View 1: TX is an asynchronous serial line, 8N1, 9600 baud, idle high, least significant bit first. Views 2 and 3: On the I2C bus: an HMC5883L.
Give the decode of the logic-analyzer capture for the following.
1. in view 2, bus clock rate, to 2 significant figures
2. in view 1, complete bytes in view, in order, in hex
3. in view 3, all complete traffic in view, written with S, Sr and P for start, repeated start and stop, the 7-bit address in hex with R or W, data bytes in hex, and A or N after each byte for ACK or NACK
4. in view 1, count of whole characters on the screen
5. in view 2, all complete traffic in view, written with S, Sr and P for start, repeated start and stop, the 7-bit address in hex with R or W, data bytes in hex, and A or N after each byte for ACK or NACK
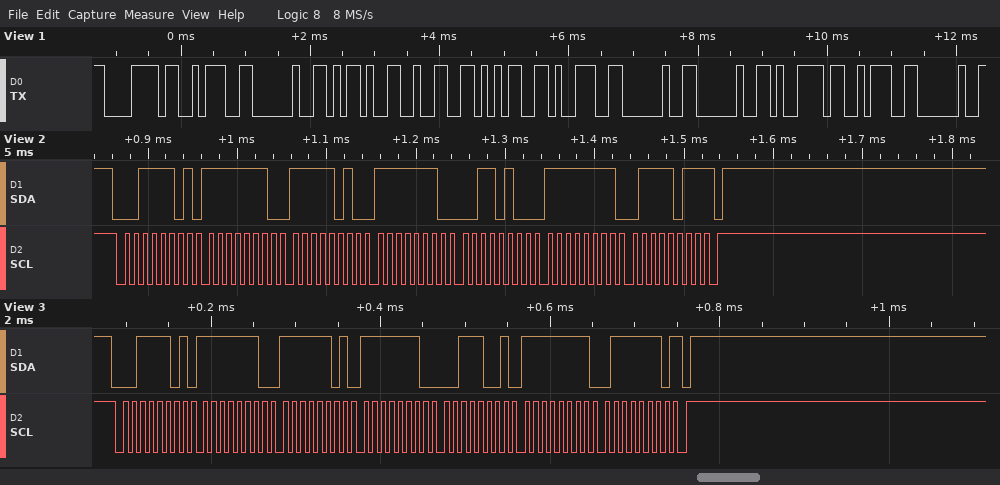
100 kHz
78 3A 20 2D 32 35 39 20 20 79 3A 20
S 1ER A FE A FD A FE A 39 A FF A 7E N P
12
S 1ER A FE A FA A FE A 34 A FF A 7B N P
